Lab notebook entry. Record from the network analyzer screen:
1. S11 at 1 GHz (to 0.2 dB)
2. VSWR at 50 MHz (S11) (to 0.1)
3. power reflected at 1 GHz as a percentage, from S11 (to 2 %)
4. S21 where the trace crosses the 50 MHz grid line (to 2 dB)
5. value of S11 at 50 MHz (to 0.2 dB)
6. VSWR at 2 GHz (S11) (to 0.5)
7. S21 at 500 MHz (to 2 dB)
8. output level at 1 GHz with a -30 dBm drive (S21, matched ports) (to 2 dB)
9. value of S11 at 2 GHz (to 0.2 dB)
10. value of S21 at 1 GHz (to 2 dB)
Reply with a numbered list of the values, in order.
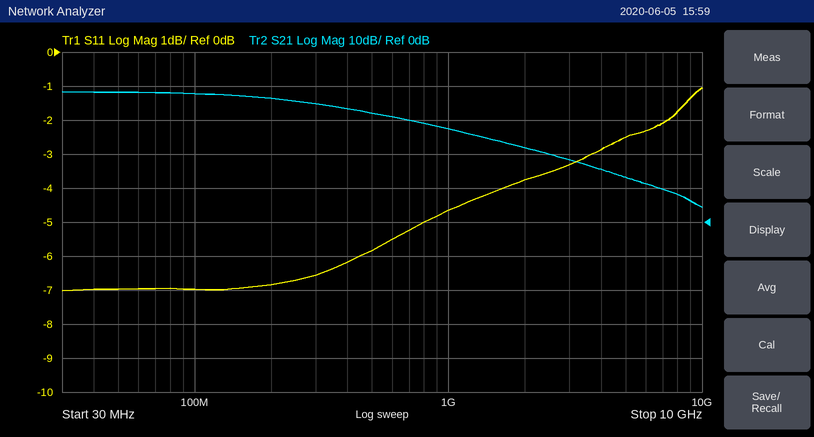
1. -4.6 dB
2. 2.6
3. 34 %
4. 38 dB
5. -7.0 dB
6. 4.5
7. 32 dB
8. -2 dBm
9. -3.8 dB
10. 28 dB
